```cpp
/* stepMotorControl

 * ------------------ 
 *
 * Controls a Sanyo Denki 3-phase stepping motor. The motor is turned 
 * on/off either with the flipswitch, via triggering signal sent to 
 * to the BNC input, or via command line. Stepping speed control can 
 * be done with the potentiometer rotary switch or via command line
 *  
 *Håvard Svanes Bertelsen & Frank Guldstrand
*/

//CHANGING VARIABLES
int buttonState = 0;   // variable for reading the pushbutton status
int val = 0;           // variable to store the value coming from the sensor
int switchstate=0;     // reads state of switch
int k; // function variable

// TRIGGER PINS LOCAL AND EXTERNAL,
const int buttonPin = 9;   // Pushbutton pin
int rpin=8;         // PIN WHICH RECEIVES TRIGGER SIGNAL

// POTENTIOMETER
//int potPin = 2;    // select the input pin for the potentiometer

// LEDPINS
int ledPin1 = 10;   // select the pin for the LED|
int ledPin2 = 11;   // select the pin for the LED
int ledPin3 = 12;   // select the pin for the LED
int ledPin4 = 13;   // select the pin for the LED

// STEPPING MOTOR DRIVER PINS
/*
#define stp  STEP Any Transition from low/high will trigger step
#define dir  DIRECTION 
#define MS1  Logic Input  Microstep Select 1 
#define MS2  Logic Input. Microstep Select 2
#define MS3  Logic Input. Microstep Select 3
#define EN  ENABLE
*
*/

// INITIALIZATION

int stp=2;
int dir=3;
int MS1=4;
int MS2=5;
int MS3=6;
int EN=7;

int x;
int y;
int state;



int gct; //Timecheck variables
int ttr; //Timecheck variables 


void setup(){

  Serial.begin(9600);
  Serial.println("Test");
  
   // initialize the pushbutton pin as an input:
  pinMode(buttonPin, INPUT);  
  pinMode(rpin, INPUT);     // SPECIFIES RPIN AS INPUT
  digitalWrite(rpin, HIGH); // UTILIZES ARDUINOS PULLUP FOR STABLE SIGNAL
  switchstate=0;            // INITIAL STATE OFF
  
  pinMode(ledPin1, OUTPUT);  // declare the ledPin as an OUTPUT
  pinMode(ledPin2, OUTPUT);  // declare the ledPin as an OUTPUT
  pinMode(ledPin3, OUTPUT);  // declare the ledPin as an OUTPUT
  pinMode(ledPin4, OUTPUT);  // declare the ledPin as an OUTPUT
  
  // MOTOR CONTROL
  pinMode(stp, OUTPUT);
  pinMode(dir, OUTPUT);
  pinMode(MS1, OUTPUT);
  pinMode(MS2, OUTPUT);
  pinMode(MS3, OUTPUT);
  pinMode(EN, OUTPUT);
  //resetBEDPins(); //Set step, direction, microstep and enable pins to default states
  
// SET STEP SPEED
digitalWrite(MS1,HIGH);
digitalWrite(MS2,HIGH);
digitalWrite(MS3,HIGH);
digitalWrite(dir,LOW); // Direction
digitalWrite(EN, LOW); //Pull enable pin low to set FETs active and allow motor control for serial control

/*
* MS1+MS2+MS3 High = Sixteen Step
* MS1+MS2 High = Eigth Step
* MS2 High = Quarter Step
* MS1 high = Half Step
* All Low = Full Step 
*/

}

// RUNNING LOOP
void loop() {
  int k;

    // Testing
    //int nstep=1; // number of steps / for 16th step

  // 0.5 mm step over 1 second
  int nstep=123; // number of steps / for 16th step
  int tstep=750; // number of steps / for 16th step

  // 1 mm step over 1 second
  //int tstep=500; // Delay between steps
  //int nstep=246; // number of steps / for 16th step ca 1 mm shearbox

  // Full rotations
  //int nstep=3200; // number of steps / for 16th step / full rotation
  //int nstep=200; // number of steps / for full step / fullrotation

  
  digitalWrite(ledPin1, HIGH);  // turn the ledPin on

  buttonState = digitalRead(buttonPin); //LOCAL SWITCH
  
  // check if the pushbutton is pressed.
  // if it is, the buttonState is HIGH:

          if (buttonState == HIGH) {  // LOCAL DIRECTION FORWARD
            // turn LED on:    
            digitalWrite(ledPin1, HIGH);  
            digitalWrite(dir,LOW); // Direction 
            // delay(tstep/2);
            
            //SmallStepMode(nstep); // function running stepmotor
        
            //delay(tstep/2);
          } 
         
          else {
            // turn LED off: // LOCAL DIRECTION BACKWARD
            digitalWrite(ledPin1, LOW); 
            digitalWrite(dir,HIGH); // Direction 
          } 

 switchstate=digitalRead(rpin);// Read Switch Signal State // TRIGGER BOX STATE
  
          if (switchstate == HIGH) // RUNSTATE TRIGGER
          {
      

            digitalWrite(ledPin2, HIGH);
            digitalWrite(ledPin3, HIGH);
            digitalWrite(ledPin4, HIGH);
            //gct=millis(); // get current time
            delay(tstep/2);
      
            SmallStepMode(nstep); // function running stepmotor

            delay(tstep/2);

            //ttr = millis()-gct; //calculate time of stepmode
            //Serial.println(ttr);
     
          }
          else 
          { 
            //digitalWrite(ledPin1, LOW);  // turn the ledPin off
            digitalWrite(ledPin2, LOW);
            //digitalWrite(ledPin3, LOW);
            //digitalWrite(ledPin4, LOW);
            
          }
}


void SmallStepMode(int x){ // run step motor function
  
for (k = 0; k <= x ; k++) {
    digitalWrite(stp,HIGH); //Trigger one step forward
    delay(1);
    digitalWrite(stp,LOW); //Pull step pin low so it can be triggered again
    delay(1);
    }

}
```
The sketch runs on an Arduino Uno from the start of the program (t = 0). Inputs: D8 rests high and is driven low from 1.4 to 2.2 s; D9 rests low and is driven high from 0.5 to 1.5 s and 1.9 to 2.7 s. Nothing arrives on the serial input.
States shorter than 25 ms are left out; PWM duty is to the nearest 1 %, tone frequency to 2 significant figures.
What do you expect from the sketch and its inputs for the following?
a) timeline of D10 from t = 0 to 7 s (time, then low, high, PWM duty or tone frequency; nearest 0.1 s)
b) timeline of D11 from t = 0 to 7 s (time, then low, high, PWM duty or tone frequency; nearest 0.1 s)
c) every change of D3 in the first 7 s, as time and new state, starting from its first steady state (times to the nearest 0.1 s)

0 s low; 1 s high; 3.2 s low
0 s high; 2 s low; 2.2 s high
0 s high; 1 s low; 3.2 s high
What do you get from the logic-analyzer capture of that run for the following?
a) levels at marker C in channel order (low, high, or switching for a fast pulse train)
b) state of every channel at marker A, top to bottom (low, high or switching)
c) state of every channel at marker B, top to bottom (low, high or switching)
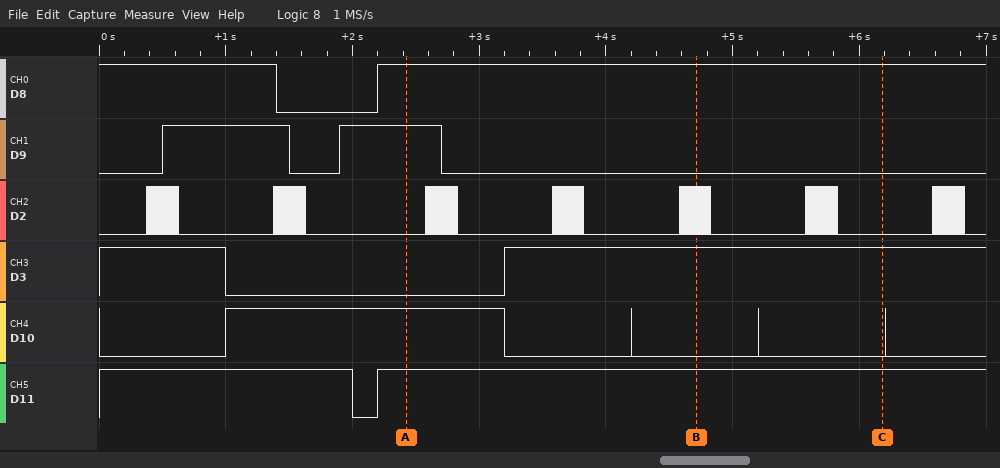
D8 high, D9 low, D2 low, D3 high, D10 low, D11 high
D8 high, D9 high, D2 low, D3 low, D10 high, D11 high
D8 high, D9 low, D2 switching, D3 high, D10 low, D11 high
